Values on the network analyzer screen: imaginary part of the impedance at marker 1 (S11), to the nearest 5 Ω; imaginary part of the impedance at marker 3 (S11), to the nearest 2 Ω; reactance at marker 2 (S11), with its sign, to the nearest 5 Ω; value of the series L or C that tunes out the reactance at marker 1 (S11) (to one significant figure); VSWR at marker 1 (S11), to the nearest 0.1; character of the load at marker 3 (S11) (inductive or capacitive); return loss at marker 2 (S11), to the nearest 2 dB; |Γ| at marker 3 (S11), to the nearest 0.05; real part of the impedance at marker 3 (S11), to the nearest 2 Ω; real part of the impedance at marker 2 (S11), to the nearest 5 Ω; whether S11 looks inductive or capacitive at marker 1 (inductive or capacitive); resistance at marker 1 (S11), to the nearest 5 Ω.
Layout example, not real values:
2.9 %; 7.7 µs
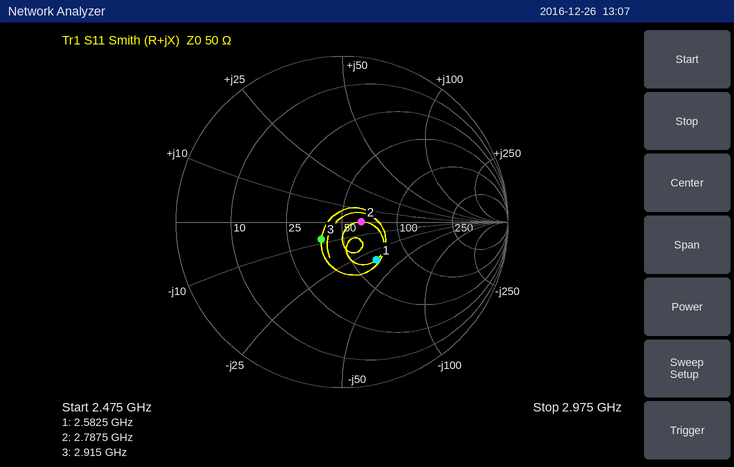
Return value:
-35 Ω; -8 Ω; 0 Ω; 2 nH; 1.9; capacitive; 18 dB; 0.15; 38 Ω; 65 Ω; capacitive; 65 Ω
